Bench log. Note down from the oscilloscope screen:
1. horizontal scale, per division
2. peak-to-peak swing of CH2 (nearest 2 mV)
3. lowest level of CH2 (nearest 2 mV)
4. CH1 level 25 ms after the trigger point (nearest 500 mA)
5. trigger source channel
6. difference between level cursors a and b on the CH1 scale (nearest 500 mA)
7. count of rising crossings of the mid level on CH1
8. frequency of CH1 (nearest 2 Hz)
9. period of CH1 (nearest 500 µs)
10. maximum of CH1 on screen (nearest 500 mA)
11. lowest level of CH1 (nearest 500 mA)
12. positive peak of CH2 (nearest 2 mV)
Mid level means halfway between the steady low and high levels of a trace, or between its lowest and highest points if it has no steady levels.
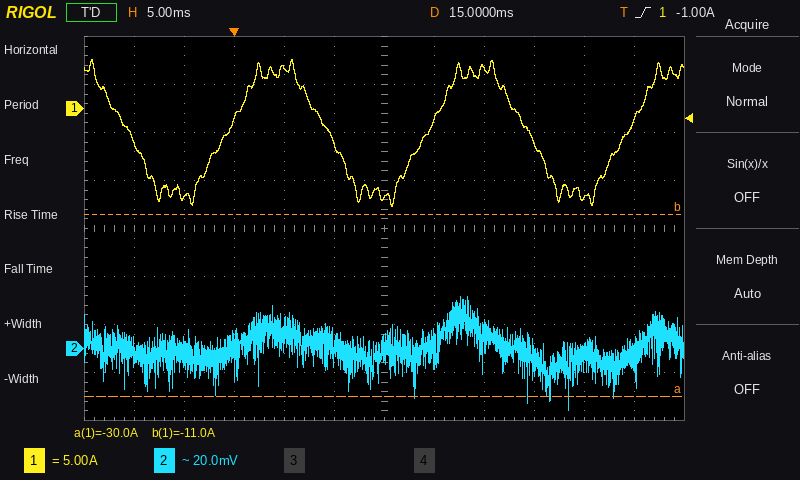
5 ms
48 mV
-26 mV
4.0 A
CH1
19.0 A
3
50 Hz
20.0 ms
5.0 A
-10.0 A
22 mV
